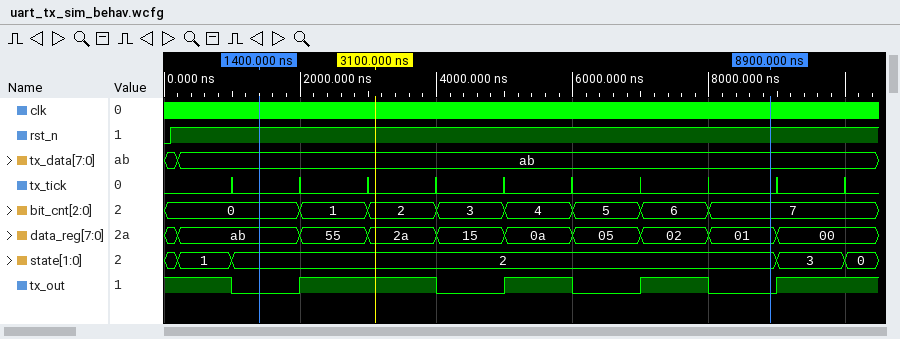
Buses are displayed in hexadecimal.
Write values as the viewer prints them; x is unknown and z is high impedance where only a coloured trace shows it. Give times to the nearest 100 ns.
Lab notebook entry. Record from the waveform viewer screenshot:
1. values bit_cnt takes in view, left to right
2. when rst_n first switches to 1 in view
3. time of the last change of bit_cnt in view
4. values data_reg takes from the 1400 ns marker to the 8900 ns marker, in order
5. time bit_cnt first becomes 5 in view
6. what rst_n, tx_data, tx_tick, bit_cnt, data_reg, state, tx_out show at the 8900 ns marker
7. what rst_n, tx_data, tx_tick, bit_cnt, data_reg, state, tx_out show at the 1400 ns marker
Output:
0, 1, 2, 3, 4, 5, 6, 7
100 ns
8000 ns
ab, 55, 2a, 15, 0a, 05, 02, 01
6000 ns
rst_n=1, tx_data=ab, tx_tick=0, bit_cnt=7, data_reg=01, state=2, tx_out=0
rst_n=1, tx_data=ab, tx_tick=0, bit_cnt=0, data_reg=ab, state=2, tx_out=0
